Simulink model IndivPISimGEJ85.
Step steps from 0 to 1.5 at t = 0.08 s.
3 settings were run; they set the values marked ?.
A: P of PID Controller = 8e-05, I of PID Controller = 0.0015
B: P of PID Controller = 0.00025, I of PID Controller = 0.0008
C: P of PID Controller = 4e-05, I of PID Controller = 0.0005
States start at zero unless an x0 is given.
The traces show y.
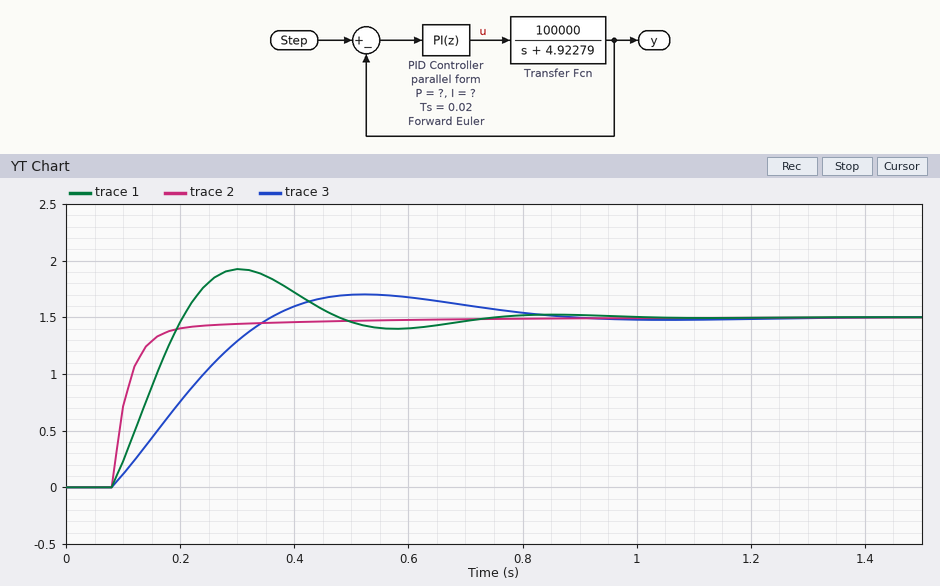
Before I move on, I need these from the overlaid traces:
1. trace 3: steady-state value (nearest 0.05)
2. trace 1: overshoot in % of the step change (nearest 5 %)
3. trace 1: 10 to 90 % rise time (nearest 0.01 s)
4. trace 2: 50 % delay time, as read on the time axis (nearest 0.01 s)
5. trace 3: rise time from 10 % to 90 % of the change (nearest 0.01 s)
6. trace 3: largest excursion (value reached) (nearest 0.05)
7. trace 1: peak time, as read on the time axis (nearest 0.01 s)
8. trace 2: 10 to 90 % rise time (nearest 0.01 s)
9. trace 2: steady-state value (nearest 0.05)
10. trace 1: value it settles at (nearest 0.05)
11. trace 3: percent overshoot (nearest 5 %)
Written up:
1.50
30 %
0.10 s
0.10 s
0.21 s
1.70
0.30 s
0.08 s
1.50
1.50
15 %
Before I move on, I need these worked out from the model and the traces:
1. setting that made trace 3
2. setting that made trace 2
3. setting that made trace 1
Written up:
C
B
A
